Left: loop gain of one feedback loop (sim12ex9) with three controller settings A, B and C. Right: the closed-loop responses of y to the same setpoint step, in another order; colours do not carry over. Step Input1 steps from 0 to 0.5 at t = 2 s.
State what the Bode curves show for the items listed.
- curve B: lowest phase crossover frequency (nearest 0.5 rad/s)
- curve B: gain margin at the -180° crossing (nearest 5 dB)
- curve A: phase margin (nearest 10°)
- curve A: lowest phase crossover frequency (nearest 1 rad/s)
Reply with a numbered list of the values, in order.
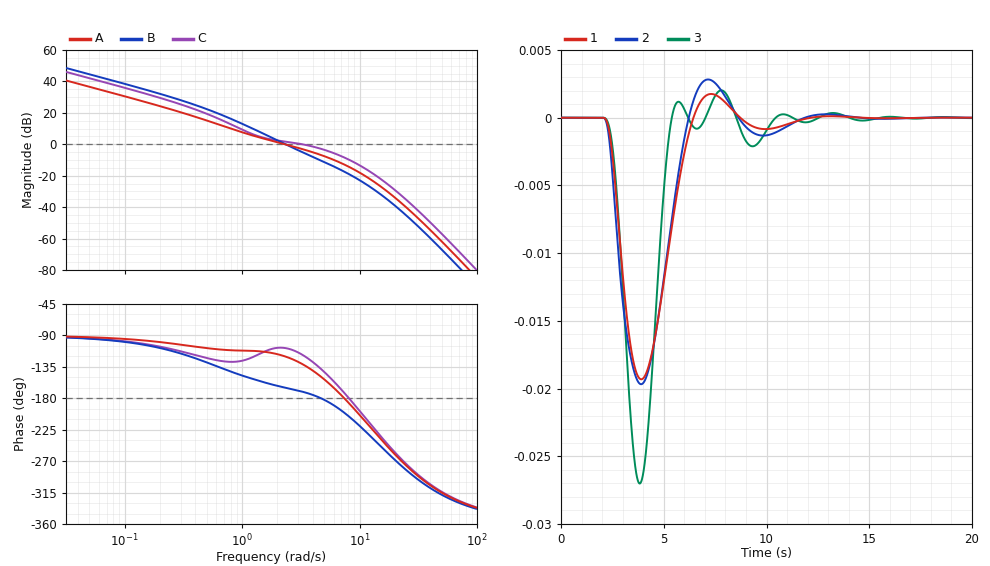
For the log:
1. 4.5 rad/s
2. 10 dB
3. 60°
4. 7 rad/s
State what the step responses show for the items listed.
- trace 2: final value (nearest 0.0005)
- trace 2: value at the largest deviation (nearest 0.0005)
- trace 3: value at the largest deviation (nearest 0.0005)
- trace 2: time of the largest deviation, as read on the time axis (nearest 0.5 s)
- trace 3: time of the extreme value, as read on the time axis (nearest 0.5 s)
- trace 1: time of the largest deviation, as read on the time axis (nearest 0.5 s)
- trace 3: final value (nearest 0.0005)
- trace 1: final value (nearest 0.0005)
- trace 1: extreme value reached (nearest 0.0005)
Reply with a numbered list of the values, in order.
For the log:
1. 0.0000
2. -0.0195
3. -0.0270
4. 4.0 s
5. 4.0 s
6. 4.0 s
7. 0.0000
8. 0.0000
9. -0.0195
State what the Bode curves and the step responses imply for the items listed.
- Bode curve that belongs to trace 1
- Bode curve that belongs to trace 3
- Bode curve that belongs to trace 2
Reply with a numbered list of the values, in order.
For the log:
1. A
2. B
3. C
